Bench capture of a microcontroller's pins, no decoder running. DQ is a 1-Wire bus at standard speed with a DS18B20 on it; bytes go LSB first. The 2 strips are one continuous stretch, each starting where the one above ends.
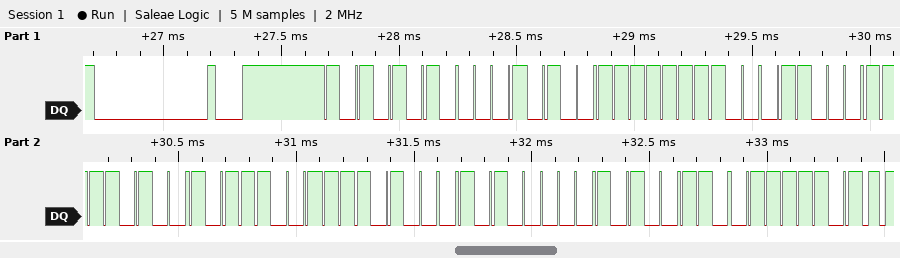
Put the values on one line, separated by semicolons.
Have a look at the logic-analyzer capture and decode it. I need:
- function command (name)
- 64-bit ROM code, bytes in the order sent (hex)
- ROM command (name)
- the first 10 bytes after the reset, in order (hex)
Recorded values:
Read Scratchpad; 28 FF 18 2F 9D 17 05 65; Match ROM; 55 28 FF 18 2F 9D 17 05 65 BE
